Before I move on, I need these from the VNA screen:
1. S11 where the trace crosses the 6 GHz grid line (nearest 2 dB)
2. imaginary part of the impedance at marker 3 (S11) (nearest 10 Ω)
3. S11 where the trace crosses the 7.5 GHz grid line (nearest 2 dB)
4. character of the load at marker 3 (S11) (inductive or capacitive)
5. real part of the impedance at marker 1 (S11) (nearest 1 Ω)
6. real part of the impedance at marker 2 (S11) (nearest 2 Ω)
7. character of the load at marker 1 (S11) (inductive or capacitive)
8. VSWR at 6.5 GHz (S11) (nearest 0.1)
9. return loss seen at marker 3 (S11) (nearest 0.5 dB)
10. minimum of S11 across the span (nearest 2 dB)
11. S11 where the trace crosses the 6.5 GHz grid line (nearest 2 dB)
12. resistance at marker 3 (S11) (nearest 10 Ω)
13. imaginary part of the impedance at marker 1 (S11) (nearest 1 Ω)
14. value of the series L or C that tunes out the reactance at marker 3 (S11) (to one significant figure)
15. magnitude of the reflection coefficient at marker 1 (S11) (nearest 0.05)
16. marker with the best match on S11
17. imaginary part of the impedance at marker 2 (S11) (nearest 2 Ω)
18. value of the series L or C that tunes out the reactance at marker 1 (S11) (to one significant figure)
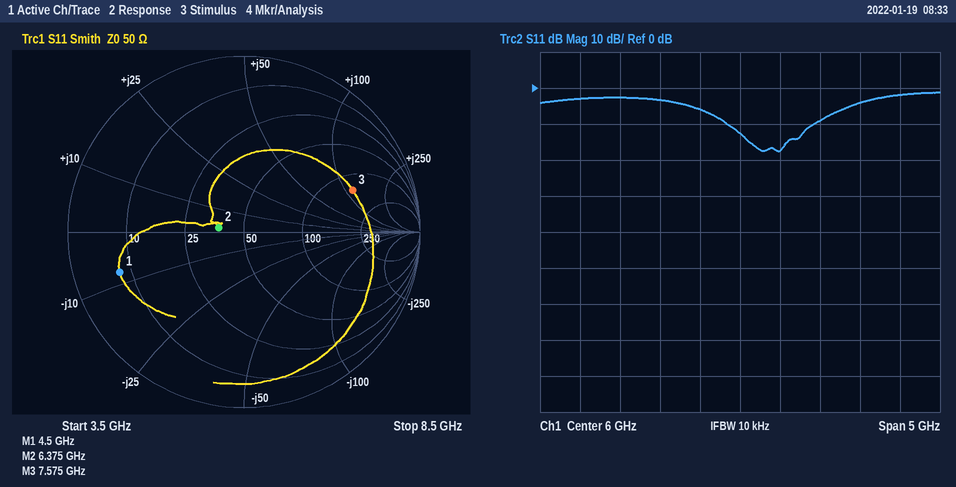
-12 dB
+120 Ω
-4 dB
inductive
8 Ω
38 Ω
capacitive
1.3
3.5 dB
-18 dB
-18 dB
140 Ω
-8 Ω
200 fF
0.75
marker 2
+2 Ω
300 pH
